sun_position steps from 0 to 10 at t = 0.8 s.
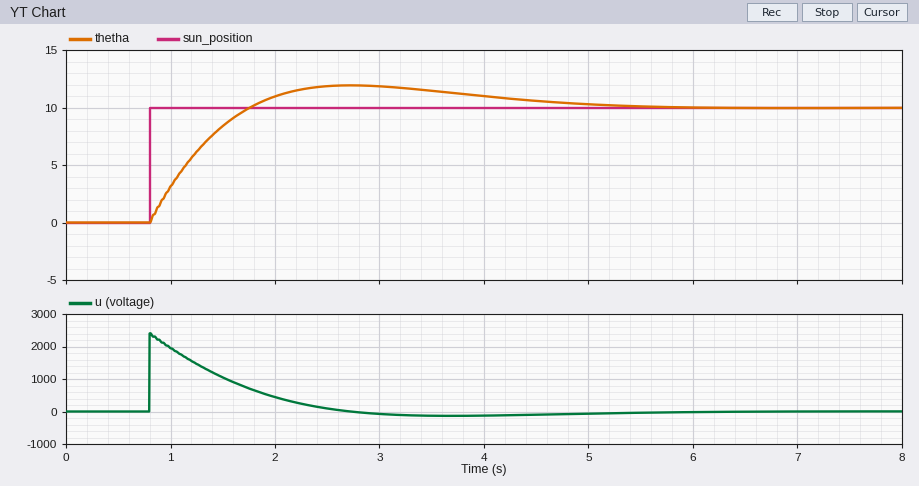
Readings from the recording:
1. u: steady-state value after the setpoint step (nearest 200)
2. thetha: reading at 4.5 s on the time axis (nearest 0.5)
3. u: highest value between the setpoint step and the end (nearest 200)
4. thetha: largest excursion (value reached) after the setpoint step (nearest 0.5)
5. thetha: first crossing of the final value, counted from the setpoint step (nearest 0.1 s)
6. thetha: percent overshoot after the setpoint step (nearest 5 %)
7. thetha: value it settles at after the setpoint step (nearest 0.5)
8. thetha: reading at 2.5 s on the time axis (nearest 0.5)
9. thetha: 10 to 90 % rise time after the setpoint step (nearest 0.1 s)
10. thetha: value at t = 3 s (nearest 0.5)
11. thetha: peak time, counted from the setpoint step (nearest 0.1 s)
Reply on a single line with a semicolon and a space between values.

0; 10.5; 2400; 12.0; 1.0 s; 20 %; 10.0; 12.0; 0.7 s; 12.0; 1.9 s
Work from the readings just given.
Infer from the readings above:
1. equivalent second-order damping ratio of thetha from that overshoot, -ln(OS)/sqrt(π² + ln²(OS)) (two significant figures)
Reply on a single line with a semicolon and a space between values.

0.46
